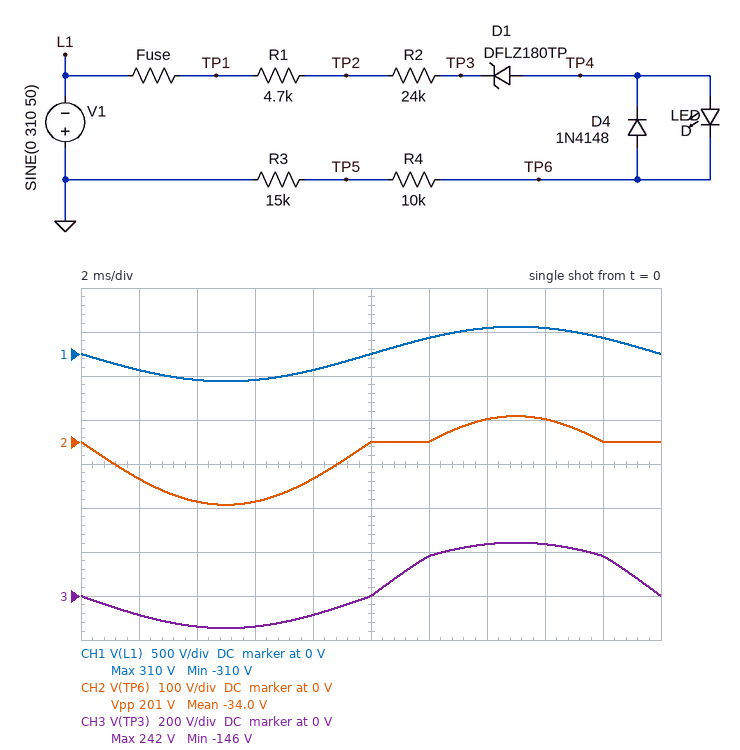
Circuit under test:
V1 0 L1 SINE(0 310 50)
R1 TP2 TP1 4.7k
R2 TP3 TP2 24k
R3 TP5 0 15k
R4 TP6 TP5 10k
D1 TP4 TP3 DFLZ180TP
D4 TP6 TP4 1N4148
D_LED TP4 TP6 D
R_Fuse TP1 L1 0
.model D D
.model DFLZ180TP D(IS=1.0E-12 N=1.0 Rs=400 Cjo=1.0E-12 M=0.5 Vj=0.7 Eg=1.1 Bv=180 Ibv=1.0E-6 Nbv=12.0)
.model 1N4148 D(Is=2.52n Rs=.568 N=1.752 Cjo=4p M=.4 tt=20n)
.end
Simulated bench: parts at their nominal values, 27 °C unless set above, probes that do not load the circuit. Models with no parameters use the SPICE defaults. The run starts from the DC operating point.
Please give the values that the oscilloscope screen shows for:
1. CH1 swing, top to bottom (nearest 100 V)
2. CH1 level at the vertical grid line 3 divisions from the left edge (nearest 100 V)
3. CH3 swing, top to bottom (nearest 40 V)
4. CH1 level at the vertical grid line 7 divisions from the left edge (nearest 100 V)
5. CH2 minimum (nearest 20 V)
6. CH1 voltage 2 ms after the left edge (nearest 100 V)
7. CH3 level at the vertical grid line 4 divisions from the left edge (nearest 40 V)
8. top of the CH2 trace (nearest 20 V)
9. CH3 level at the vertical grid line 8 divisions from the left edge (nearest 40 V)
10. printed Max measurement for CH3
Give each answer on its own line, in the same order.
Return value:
600 V
-300 V
400 V
300 V
-140 V
-200 V
-80 V
60 V
240 V
242 V
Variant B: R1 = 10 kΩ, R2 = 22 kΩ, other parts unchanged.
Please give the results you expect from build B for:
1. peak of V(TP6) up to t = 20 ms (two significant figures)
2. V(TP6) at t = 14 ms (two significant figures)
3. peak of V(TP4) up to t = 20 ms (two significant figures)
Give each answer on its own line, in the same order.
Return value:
55 V
49 V
56 V
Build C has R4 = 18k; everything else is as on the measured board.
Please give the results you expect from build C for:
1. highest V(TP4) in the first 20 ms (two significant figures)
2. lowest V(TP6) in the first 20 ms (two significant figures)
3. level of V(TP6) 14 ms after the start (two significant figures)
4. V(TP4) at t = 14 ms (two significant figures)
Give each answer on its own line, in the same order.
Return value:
68 V
-160 V
59 V
60 V
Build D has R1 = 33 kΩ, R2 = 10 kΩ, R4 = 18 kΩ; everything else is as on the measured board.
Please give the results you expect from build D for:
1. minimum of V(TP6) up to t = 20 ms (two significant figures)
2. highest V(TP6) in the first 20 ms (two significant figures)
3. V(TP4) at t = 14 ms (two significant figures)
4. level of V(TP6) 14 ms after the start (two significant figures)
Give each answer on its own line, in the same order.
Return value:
-130 V
55 V
49 V
48 V
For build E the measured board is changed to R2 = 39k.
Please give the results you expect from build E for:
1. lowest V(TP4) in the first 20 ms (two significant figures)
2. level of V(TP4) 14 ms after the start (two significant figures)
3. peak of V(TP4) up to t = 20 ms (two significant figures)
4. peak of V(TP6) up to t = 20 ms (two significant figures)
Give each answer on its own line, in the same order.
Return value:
-110 V
41 V
47 V
46 V
